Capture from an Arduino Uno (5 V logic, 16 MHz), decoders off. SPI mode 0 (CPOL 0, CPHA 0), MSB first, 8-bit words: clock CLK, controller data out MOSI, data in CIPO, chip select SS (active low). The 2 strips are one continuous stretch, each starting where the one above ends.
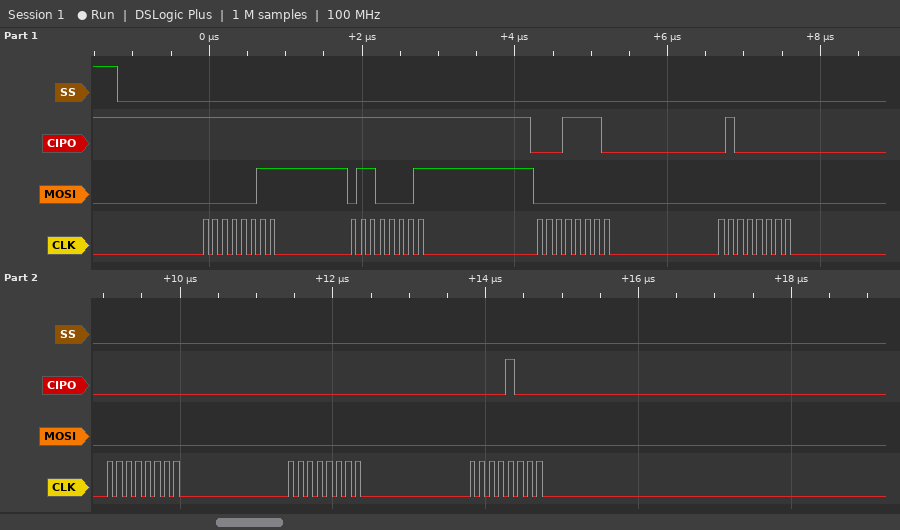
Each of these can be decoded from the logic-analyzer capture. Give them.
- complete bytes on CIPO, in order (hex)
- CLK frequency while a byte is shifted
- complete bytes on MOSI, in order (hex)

FF FF 1E 40 00 00 08
8 MHz
03 61 00 00 00 00 00
